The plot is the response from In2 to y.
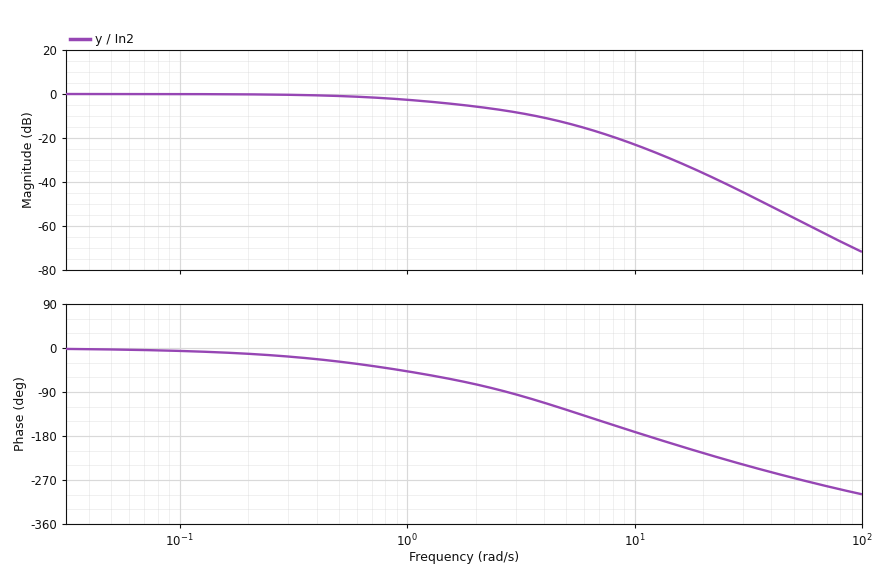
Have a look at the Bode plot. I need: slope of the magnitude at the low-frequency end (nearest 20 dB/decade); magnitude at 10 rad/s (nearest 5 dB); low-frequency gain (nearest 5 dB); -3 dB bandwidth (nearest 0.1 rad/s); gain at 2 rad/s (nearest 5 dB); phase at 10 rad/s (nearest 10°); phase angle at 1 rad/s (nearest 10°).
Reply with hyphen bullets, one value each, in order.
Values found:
- 0 dB/decade
- -25 dB
- 0 dB
- 1.1 rad/s
- -5 dB
- -170°
- -50°
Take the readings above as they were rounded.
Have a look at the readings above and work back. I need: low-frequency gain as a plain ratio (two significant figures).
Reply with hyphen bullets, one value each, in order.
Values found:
- 1.0
